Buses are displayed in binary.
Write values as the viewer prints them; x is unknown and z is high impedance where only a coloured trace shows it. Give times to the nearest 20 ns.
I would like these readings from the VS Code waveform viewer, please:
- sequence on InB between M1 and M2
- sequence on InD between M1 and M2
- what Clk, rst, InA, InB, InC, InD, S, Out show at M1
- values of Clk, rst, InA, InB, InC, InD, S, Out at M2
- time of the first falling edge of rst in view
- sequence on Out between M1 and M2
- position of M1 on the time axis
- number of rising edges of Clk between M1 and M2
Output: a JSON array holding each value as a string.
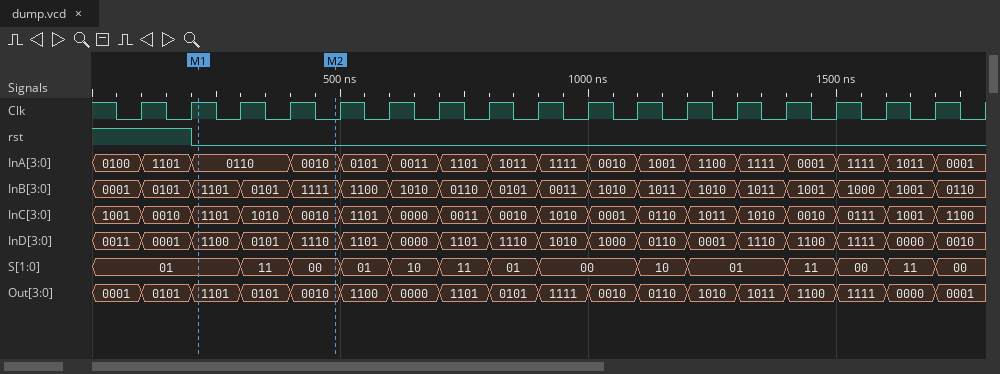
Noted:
["1101, 0101, 1111", "1100, 0101, 1110", "Clk=1, rst=0, InA=0110, InB=1101, InC=1101, InD=1100, S=01, Out=1101", "Clk=0, rst=0, InA=0010, InB=1111, InC=0010, InD=1110, S=00, Out=0010", "200 ns", "1101, 0101, 0010", "220 ns", "2"]
